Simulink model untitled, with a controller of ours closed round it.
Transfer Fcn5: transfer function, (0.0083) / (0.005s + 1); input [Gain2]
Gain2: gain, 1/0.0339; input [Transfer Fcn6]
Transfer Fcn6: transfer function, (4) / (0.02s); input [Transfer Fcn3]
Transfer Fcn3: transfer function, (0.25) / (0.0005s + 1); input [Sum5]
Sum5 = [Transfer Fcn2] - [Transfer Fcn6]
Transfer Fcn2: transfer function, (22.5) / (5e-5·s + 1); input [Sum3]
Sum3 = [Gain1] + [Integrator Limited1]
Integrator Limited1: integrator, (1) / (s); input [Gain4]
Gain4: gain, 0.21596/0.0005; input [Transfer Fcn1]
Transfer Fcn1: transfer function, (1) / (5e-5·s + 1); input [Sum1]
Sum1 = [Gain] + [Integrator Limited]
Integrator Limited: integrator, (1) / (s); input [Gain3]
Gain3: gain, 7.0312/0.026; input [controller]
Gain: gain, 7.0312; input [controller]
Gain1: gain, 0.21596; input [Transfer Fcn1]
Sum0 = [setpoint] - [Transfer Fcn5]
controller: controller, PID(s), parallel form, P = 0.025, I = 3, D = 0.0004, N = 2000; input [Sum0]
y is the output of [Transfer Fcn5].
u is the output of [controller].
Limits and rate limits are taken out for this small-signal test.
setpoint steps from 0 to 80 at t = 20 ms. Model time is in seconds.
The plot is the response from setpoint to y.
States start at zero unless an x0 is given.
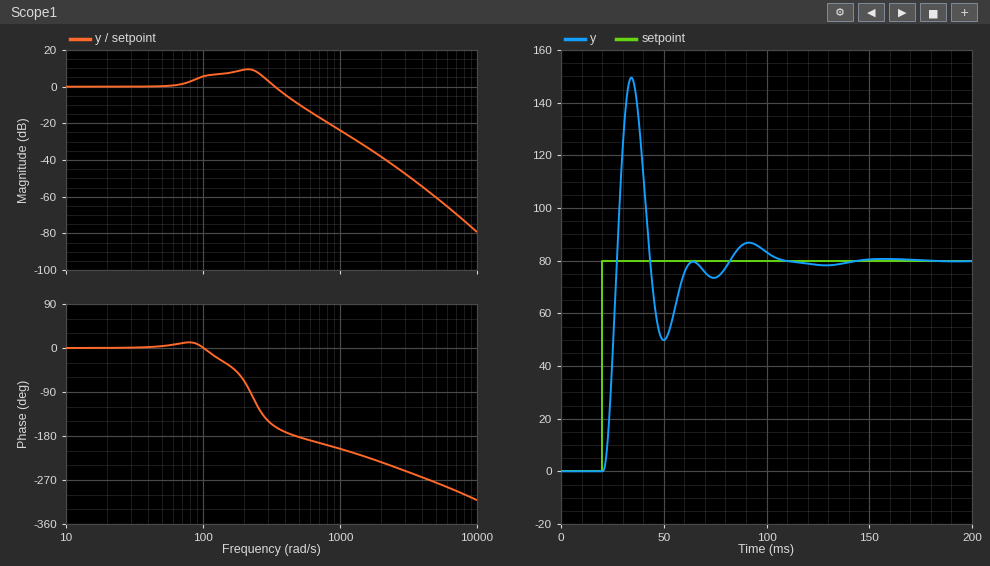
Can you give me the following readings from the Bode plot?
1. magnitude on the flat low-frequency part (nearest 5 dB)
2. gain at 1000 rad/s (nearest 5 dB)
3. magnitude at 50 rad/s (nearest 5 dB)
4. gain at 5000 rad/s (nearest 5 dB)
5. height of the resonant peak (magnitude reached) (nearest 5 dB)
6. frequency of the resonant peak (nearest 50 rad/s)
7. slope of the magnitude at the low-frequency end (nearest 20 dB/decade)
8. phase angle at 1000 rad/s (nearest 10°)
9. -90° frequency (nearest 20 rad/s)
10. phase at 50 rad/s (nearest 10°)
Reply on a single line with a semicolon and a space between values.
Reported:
0 dB; -25 dB; 0 dB; -60 dB; 10 dB; 200 rad/s; 0 dB/decade; -210°; 220 rad/s; 0°
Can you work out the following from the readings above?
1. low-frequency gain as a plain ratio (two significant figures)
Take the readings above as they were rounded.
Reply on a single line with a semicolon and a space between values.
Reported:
1.0
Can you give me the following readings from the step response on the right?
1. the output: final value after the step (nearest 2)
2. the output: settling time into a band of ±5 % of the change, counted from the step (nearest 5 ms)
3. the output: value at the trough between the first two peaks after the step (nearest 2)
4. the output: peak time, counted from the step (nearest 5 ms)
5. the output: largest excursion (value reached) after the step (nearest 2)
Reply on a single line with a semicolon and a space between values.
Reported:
80; 80 ms; 50; 15 ms; 150
